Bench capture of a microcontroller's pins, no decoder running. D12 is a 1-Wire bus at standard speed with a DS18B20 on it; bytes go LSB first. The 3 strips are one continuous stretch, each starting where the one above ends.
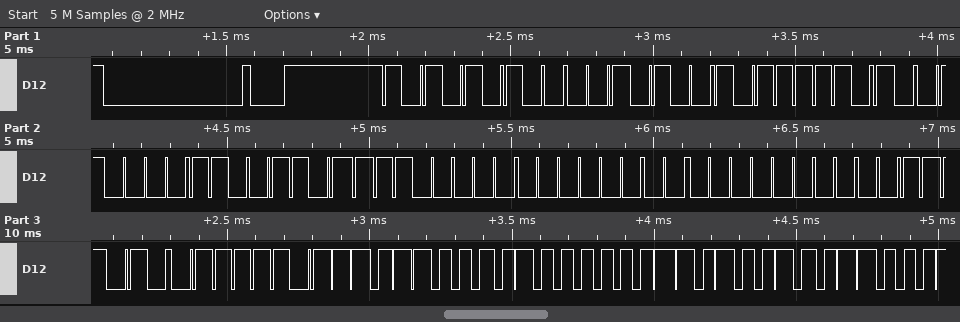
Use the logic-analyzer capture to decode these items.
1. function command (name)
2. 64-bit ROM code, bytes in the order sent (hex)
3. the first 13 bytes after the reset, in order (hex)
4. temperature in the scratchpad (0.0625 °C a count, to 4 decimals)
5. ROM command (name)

Read Scratchpad
28 7D 09 B3 07 00 00 5C
55 28 7D 09 B3 07 00 00 5C BE 1B 02 4B
33.6875 °C
Match ROM
